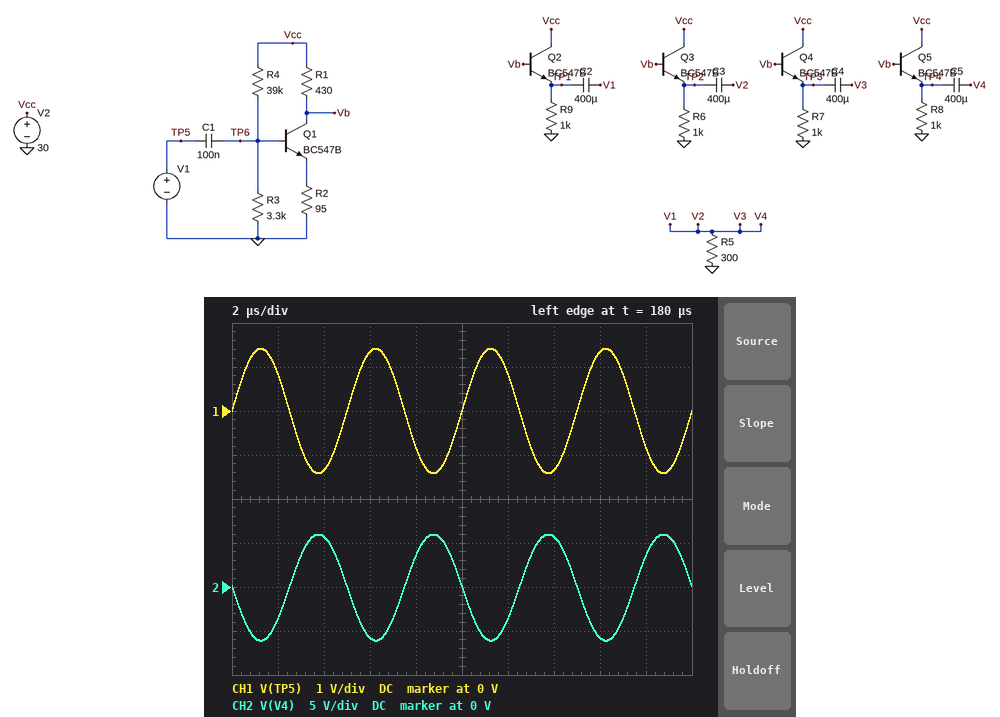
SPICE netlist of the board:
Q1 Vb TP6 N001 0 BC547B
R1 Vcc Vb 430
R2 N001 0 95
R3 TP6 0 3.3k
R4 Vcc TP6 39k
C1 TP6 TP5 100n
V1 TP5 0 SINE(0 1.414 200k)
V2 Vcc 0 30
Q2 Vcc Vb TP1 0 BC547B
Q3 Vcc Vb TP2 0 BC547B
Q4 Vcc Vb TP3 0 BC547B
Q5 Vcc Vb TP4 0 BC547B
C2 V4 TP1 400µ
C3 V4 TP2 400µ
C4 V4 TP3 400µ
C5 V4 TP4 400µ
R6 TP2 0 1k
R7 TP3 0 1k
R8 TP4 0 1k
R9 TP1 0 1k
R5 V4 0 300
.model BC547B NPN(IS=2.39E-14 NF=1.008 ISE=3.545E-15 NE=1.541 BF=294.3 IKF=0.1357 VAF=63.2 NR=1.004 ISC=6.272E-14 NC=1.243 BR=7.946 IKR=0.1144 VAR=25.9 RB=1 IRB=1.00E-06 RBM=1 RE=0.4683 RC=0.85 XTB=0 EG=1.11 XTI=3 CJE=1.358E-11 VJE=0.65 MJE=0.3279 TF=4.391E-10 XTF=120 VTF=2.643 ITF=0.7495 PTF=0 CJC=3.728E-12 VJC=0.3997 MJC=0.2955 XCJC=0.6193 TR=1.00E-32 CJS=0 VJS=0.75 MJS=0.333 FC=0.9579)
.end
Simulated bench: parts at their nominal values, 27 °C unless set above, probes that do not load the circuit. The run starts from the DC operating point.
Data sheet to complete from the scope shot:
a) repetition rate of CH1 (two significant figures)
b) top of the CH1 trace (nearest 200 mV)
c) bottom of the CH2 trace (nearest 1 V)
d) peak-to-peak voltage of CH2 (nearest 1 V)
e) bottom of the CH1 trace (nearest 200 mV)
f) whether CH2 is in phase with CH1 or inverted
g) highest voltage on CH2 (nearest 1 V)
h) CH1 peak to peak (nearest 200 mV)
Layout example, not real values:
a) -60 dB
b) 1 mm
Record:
a) 200 kHz
b) 1.4 V
c) -6 V
d) 12 V
e) -1.4 V
f) inverted
g) 6 V
h) 2.8 V
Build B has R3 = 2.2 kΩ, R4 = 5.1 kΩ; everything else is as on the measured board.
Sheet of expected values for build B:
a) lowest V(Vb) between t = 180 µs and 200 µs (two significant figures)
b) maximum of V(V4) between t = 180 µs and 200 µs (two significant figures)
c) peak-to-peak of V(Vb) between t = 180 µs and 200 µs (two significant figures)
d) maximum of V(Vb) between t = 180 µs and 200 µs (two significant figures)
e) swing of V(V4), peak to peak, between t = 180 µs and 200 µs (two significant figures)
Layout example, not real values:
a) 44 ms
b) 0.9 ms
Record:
a) 5.6 V
b) 8.9 V
c) 9.1 V
d) 15 V
e) 9.0 V
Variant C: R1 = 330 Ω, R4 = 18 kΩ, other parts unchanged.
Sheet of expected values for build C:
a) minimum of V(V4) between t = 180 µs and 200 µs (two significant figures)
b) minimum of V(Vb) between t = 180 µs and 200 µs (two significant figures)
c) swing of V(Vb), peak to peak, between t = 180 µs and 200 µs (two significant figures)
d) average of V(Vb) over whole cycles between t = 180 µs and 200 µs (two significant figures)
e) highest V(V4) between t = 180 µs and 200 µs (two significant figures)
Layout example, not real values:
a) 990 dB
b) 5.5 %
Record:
a) -4.7 V
b) 13 V
c) 9.5 V
d) 18 V
e) 4.8 V
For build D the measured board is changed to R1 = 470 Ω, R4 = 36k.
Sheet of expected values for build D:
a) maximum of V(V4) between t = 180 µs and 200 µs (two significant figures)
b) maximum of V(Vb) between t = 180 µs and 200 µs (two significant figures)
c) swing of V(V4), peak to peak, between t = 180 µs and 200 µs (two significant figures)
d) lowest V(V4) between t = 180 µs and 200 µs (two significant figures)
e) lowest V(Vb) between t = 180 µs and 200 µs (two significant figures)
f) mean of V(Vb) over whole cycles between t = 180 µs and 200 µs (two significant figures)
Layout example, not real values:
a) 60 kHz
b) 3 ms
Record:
a) 6.6 V
b) 28 V
c) 13 V
d) -6.7 V
e) 15 V
f) 22 V
